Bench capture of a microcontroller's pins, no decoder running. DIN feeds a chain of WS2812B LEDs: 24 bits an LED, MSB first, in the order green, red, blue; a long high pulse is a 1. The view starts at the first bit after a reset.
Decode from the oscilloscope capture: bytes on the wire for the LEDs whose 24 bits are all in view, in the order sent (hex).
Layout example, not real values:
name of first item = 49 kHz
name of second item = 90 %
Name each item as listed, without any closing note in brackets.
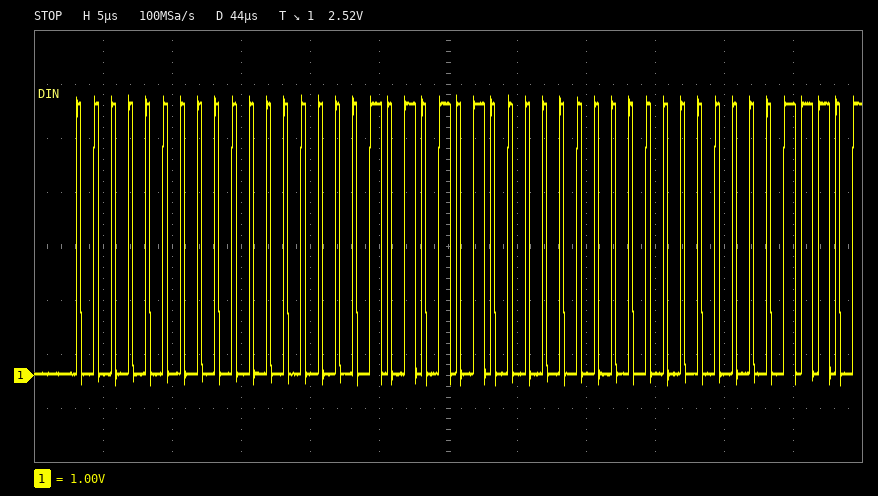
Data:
bytes on the wire for the LEDs whose 24 bits are all in view, in the order sent = 00 00 55
